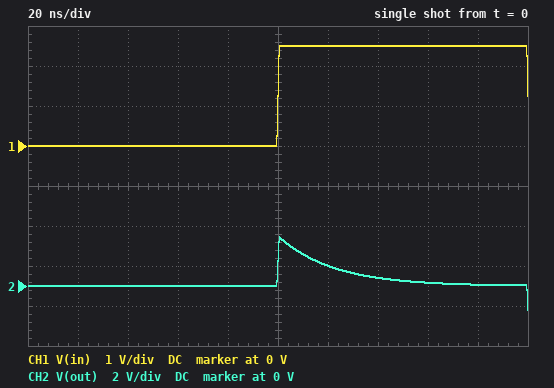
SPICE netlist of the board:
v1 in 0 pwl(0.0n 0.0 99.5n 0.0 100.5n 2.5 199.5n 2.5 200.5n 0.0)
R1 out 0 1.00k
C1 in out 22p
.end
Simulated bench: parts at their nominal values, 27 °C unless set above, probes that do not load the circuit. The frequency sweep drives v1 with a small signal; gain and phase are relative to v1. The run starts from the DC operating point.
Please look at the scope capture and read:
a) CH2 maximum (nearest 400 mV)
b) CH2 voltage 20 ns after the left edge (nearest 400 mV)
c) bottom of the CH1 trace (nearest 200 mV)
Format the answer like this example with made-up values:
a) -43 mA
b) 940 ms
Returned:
a) 2.4 V
b) 0 V
c) 0 V
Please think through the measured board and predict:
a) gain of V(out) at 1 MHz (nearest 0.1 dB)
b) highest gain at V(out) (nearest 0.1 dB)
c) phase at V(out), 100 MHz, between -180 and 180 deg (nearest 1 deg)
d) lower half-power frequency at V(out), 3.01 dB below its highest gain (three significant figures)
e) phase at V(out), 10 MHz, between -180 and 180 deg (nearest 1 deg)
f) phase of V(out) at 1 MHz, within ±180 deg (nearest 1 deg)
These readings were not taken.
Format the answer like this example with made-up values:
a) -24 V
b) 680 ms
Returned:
a) -17.3 dB
b) 0 dB
c) 4 deg
d) 7.23 MHz
e) 36 deg
f) 82 deg
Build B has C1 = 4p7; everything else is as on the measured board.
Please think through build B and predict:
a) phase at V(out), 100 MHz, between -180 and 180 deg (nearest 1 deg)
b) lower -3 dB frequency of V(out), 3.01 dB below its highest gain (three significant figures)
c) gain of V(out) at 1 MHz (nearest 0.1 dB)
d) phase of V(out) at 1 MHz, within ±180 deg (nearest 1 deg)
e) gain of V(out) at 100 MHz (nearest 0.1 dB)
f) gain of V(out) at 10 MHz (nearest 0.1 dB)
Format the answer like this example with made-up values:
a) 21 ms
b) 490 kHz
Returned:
a) 19 deg
b) 33.9 MHz
c) -30.6 dB
d) 88 deg
e) -0.5 dB
f) -11.0 dB
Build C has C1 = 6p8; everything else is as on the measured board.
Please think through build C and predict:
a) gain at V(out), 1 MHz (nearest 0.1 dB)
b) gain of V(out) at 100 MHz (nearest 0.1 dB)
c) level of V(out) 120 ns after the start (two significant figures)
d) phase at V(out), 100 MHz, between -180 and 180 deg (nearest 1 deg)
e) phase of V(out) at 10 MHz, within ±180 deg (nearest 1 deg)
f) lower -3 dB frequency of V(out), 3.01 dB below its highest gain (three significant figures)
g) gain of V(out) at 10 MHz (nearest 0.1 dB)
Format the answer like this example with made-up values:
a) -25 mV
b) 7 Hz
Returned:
a) -27.4 dB
b) -0.2 dB
c) 130 mV
d) 13 deg
e) 67 deg
f) 23.4 MHz
g) -8.1 dB
